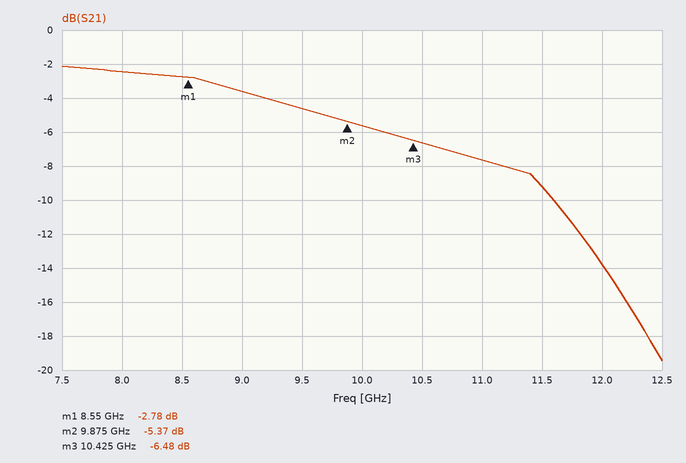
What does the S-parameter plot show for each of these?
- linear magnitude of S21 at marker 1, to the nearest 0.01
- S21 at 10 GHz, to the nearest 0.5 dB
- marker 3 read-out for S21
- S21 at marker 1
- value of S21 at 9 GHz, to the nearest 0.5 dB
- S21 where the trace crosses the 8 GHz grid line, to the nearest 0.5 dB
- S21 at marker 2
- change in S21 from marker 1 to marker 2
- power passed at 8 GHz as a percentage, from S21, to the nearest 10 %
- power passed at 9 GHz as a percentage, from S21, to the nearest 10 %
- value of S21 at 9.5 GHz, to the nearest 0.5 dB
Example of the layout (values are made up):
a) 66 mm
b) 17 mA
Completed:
a) 0.73
b) -5.5 dB
c) -6.48 dB
d) -2.78 dB
e) -3.5 dB
f) -2.5 dB
g) -5.37 dB
h) -2.59 dB
i) 60 %
j) 40 %
k) -4.5 dB
